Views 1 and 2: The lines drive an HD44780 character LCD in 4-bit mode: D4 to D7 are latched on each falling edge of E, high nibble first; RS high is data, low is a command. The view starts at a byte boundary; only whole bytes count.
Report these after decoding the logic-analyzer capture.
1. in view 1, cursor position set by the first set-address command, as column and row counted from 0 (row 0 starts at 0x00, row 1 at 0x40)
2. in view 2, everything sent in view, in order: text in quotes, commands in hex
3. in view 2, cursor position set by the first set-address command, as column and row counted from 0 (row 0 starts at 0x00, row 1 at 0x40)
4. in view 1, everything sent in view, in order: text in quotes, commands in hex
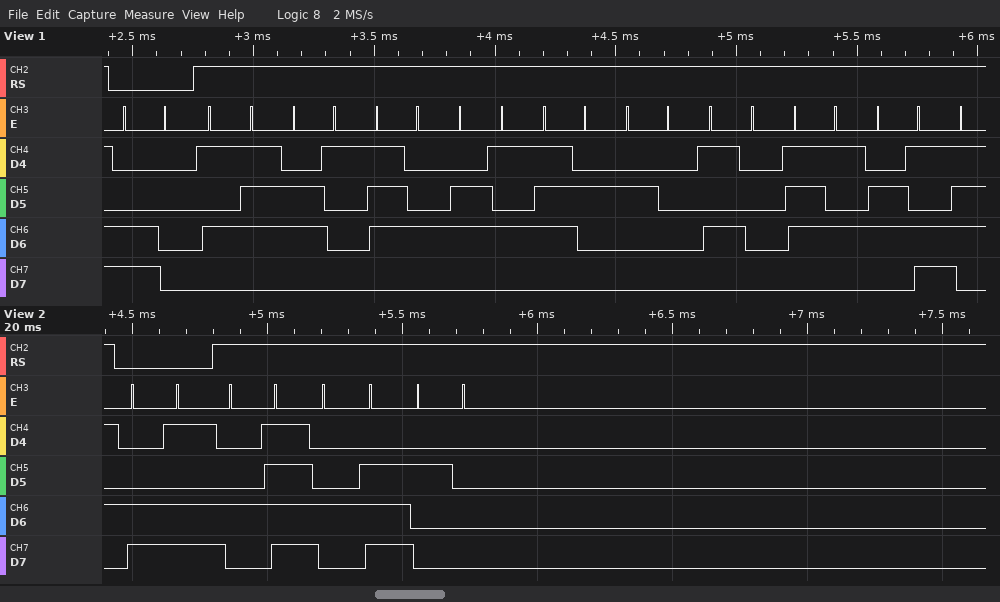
column 0, row 1
0xCD "ON "
column 13, row 1
0xC0 "Water Pum"
